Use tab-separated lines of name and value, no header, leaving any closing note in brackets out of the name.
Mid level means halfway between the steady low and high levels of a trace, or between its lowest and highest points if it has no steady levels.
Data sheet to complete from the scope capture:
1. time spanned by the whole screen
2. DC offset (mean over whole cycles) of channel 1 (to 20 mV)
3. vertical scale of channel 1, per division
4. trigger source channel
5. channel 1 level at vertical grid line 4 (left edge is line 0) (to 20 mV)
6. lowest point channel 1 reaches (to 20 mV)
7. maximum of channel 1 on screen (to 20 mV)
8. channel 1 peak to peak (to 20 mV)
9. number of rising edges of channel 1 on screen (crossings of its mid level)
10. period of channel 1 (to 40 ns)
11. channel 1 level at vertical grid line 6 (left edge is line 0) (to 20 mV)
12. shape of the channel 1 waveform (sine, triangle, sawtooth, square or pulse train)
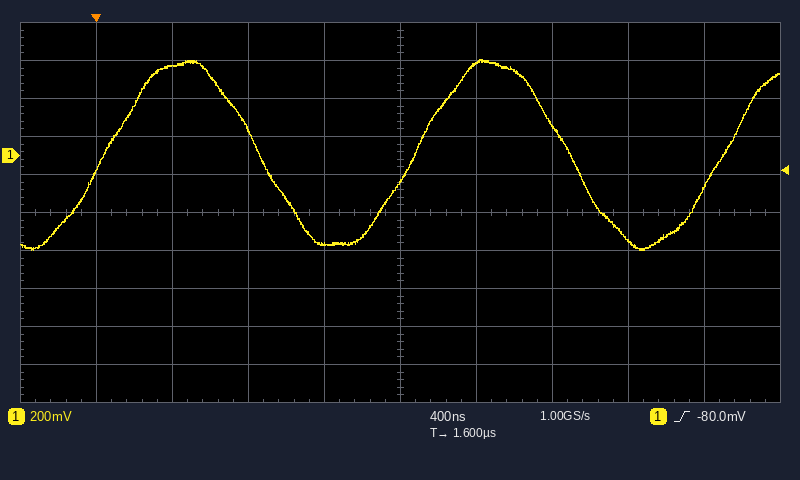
time spanned by the whole screen	4 µs
DC offset (mean over whole cycles) of channel 1	0 mV
vertical scale of channel 1, per division	200 mV
trigger source channel	channel 1
channel 1 level at vertical grid line 4 (left edge is line 0)	-460 mV
lowest point channel 1 reaches	-500 mV
maximum of channel 1 on screen	500 mV
channel 1 peak to peak	1.00 V
number of rising edges of channel 1 on screen	3
period of channel 1	1.64 µs
channel 1 level at vertical grid line 6 (left edge is line 0)	480 mV
shape of the channel 1 waveform	sine
